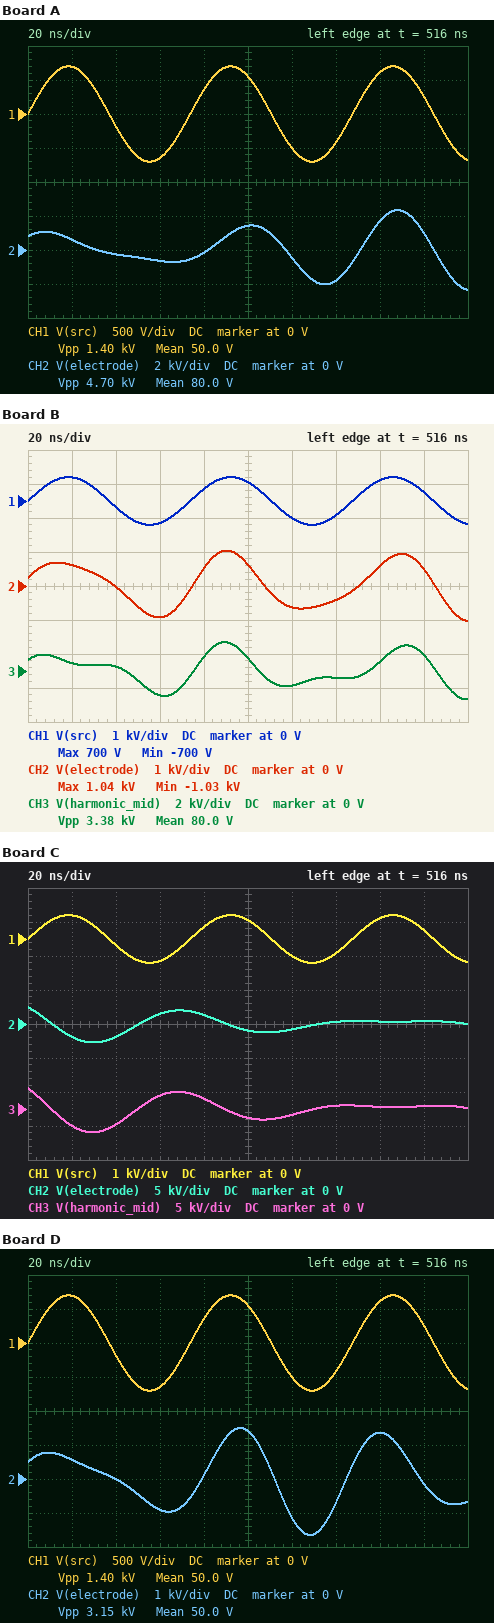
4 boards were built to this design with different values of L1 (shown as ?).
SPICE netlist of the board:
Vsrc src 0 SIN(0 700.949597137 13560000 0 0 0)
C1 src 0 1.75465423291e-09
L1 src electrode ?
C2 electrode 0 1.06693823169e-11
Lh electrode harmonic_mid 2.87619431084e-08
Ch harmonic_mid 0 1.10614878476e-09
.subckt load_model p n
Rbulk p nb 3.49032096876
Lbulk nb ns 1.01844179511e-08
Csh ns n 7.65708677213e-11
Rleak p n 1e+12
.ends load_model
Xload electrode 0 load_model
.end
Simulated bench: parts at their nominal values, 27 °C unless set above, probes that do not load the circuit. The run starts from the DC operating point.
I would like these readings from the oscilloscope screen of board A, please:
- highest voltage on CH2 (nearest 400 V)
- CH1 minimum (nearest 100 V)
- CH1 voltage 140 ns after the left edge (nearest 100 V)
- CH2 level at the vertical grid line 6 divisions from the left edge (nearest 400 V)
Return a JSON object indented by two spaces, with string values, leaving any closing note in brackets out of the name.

{
  "highest voltage on CH2": "2.4 kV",
  "CH1 minimum": "-700 V",
  "CH1 voltage 140 ns after the left edge": "-400 V",
  "CH2 level at the vertical grid line 6 divisions from the left edge": "-400 V"
}
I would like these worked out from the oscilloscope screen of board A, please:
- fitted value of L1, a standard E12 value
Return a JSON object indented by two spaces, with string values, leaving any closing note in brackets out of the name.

{
  "fitted value of L1, a standard E12 value": "47 nH"
}
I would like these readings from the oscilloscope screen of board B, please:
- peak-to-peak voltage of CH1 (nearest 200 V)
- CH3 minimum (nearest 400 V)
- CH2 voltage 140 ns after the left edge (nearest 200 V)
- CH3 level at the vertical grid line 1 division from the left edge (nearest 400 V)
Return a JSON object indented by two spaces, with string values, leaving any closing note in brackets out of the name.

{
  "peak-to-peak voltage of CH1": "1.4 kV",
  "CH3 minimum": "-1.6 kV",
  "CH2 voltage 140 ns after the left edge": "-400 V",
  "CH3 level at the vertical grid line 1 division from the left edge": "400 V"
}
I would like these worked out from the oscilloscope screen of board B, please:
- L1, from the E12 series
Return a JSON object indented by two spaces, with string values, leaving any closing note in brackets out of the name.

{
  "L1, from the E12 series": "15 nH"
}
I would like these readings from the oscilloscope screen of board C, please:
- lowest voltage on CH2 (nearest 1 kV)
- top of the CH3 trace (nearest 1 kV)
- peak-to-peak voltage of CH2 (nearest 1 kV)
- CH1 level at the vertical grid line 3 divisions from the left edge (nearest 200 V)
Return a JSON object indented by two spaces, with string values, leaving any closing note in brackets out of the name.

{
  "lowest voltage on CH2": "-3 kV",
  "top of the CH3 trace": "3 kV",
  "peak-to-peak voltage of CH2": "5 kV",
  "CH1 level at the vertical grid line 3 divisions from the left edge": "-600 V"
}
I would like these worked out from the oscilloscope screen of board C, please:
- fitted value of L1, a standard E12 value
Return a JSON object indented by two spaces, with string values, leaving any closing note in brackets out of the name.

{
  "fitted value of L1, a standard E12 value": "120 nH"
}
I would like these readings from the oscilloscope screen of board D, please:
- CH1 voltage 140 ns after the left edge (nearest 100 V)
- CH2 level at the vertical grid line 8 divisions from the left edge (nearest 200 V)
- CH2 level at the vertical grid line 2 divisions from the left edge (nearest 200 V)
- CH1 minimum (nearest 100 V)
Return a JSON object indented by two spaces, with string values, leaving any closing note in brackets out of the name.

{
  "CH1 voltage 140 ns after the left edge": "-400 V",
  "CH2 level at the vertical grid line 8 divisions from the left edge": "1.4 kV",
  "CH2 level at the vertical grid line 2 divisions from the left edge": "0 V",
  "CH1 minimum": "-700 V"
}
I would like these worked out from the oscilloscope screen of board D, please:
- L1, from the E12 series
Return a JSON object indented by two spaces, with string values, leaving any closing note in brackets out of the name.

{
  "L1, from the E12 series": "33 nH"
}
